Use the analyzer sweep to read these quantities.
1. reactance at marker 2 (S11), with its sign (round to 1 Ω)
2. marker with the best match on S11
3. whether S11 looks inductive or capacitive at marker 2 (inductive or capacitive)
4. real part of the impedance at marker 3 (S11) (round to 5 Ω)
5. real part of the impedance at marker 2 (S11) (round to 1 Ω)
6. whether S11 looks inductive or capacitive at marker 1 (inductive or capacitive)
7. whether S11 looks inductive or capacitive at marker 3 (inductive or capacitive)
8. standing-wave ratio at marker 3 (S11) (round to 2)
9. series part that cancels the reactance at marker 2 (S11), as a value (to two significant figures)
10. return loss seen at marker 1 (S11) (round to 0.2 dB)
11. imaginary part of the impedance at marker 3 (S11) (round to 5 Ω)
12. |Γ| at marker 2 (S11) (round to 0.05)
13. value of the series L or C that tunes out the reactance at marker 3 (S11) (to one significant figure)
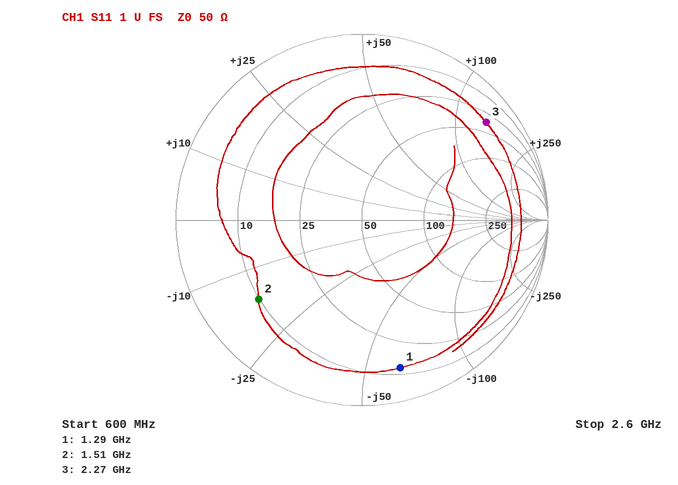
-16 Ω
marker 2
capacitive
35 Ω
10 Ω
capacitive
inductive
12
1.7 nH
1.8 dB
+135 Ω
0.70
500 fF
